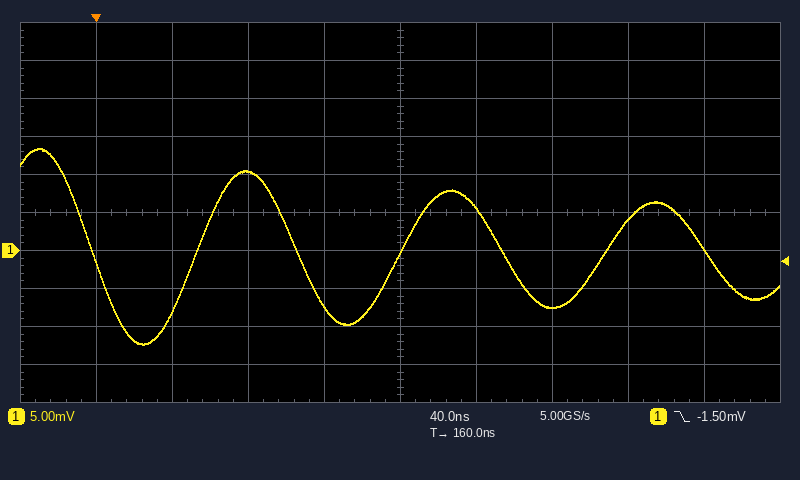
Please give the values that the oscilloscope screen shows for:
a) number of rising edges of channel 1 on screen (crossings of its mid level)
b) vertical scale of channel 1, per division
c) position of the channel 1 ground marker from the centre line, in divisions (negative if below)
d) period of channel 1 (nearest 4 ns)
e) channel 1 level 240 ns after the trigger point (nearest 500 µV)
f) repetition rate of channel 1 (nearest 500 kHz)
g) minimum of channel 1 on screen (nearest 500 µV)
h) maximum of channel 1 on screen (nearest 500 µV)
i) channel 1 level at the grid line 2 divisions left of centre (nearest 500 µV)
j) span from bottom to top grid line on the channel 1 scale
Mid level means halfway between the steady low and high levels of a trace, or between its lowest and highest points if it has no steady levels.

3
5 mV
-1.0 div
108 ns
-7.5 mV
9.5 MHz
-12.5 mV
13.5 mV
10.5 mV
50 mV
